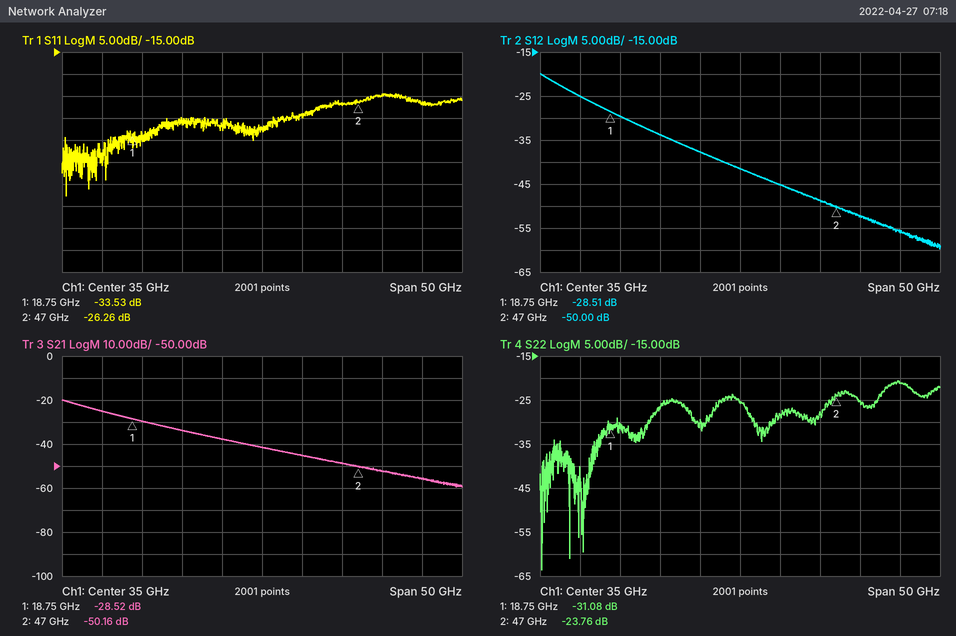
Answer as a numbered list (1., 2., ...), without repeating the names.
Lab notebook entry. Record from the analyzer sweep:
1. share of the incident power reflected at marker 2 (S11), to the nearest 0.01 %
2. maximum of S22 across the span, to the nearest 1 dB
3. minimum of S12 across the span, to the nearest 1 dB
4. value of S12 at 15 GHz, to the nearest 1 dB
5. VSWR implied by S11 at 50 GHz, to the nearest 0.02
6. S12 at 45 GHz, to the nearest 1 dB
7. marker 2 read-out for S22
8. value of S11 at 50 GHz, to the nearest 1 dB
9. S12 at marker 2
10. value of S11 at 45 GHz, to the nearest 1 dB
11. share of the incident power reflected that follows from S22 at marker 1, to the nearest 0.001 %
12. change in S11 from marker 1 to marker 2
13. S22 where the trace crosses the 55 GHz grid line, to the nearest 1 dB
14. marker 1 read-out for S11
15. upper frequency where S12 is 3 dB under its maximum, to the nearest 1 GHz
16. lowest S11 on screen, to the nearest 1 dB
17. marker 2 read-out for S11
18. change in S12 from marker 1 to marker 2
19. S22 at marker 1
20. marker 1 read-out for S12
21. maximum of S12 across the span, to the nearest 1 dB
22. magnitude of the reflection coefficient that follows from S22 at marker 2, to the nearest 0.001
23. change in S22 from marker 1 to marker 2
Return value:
1. 0.24 %
2. -21 dB
3. -60 dB
4. -25 dB
5. 1.12
6. -49 dB
7. -23.76 dB
8. -25 dB
9. -50.00 dB
10. -27 dB
11. 0.078 %
12. 7.27 dB
13. -21 dB
14. -33.53 dB
15. 13 GHz
16. -48 dB
17. -26.26 dB
18. -21.49 dB
19. -31.08 dB
20. -28.51 dB
21. -20 dB
22. 0.065
23. 7.32 dB
